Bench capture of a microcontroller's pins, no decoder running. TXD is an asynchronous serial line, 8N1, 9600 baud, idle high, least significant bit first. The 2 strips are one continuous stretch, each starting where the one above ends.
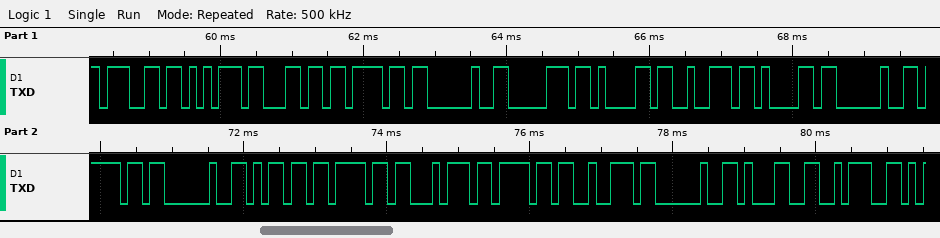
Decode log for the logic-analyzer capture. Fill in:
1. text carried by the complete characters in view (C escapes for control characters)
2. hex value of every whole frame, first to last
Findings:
"gulo para o motor 1:"
67 75 6C 6F 20 70 61 72 61 20 6F 20 6D 6F 74 6F 72 20 31 3A
